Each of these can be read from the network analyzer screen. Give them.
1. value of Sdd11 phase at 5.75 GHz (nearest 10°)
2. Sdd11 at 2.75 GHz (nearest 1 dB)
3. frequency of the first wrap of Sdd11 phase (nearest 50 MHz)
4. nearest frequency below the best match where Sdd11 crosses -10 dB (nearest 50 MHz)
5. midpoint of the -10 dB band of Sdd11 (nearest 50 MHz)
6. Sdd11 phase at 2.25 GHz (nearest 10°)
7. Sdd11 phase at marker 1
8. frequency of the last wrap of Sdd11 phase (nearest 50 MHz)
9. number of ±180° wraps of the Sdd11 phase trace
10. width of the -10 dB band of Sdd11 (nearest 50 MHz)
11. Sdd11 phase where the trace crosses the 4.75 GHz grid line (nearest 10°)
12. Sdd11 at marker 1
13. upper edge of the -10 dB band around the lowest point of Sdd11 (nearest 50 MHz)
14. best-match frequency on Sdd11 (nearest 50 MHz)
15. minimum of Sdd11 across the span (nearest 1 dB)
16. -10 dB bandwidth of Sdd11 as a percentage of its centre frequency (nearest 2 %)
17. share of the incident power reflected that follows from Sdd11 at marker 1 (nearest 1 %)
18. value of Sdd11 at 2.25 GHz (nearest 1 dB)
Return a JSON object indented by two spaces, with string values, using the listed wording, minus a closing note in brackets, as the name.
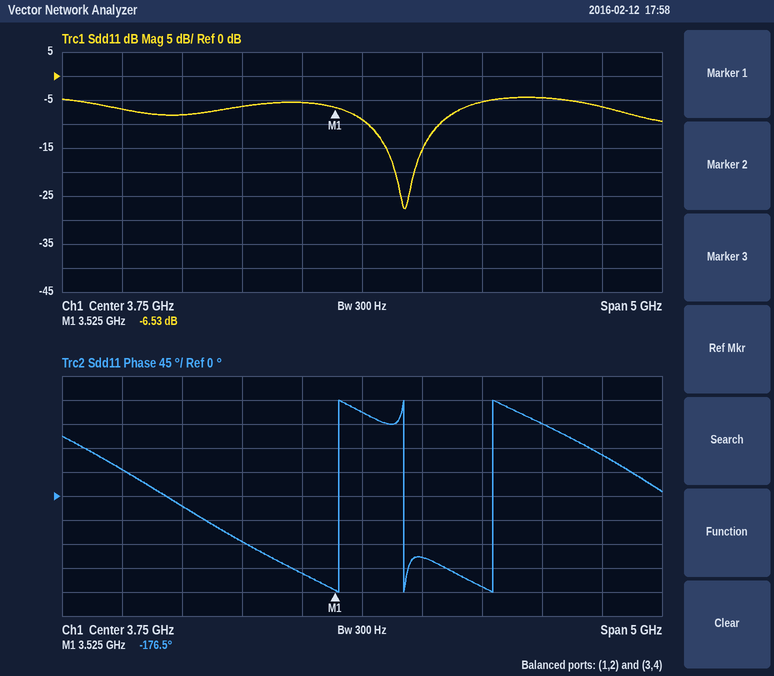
{
  "value of Sdd11 phase at 5.75 GHz": "80°",
  "Sdd11 at 2.75 GHz": "-6 dB",
  "frequency of the first wrap of Sdd11 phase": "3.55 GHz",
  "nearest frequency below the best match where Sdd11 crosses -10 dB": "3.80 GHz",
  "midpoint of the -10 dB band of Sdd11": "4.10 GHz",
  "Sdd11 phase at 2.25 GHz": "-20°",
  "Sdd11 phase at marker 1": "-176.5°",
  "frequency of the last wrap of Sdd11 phase": "4.85 GHz",
  "number of ±180° wraps of the Sdd11 phase trace": "3",
  "width of the -10 dB band of Sdd11": "600 MHz",
  "Sdd11 phase where the trace crosses the 4.75 GHz grid line": "-170°",
  "Sdd11 at marker 1": "-6.53 dB",
  "upper edge of the -10 dB band around the lowest point of Sdd11": "4.40 GHz",
  "best-match frequency on Sdd11": "4.10 GHz",
  "minimum of Sdd11 across the span": "-28 dB",
  "-10 dB bandwidth of Sdd11 as a percentage of its centre frequency": "14 %",
  "share of the incident power reflected that follows from Sdd11 at marker 1": "22 %",
  "value of Sdd11 at 2.25 GHz": "-8 dB"
}
